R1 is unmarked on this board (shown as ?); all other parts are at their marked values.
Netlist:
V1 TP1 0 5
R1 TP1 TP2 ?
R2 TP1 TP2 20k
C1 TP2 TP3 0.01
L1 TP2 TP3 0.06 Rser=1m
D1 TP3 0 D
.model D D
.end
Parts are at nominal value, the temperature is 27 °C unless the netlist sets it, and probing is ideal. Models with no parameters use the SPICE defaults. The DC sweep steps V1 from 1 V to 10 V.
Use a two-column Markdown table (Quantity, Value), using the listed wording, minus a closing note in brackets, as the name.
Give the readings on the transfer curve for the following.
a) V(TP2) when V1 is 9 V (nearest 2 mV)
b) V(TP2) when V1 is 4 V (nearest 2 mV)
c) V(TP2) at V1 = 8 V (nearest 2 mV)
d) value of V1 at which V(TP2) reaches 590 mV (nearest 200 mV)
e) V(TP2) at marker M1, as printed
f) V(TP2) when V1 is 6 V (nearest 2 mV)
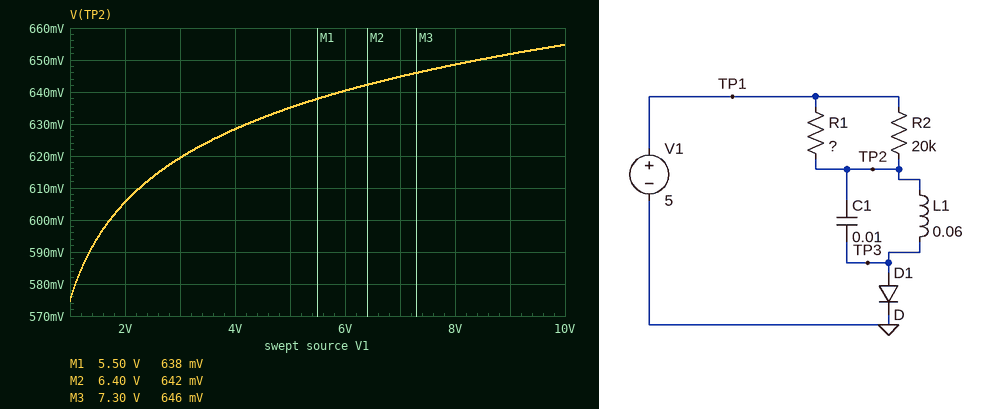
| Quantity | Value |
|---|---|
| V(TP2) when V1 is 9 V | 652 mV |
| V(TP2) when V1 is 4 V | 628 mV |
| V(TP2) at V1 = 8 V | 648 mV |
| value of V1 at which V(TP2) reaches 590 mV | 1.4 V |
| V(TP2) at marker M1, as printed | 638 mV |
| V(TP2) when V1 is 6 V | 640 mV |
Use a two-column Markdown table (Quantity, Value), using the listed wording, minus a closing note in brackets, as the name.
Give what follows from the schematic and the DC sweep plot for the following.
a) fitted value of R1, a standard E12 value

| Quantity | Value |
|---|---|
| fitted value of R1, a standard E12 value | 18 kΩ |
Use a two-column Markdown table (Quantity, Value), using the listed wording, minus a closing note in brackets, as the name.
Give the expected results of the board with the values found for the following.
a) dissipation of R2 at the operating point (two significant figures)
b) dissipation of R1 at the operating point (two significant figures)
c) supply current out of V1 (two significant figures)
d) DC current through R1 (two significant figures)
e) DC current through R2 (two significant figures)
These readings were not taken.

| Quantity | Value |
|---|---|
| dissipation of R2 at the operating point | 950 µW |
| dissipation of R1 at the operating point | 1.1 mW |
| supply current out of V1 | 460 µA |
| DC current through R1 | 240 µA |
| DC current through R2 | 220 µA |
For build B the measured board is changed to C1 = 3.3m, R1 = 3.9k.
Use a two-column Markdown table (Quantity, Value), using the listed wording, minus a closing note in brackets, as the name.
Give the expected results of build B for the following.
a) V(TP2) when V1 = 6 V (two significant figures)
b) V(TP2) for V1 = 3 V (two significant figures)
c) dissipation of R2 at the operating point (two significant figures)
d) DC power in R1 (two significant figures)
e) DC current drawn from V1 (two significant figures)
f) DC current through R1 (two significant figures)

| Quantity | Value |
|---|---|
| V(TP2) when V1 = 6 V | 670 mV |
| V(TP2) for V1 = 3 V | 650 mV |
| dissipation of R2 at the operating point | 940 µW |
| DC power in R1 | 4.8 mW |
| DC current drawn from V1 | 1.3 mA |
| DC current through R1 | 1.1 mA |
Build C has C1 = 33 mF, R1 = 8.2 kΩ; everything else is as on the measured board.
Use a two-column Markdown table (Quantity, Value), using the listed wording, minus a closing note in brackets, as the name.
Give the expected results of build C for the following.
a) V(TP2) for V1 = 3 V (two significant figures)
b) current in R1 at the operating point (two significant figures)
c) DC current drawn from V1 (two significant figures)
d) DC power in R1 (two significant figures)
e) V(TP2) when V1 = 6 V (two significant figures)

| Quantity | Value |
|---|---|
| V(TP2) for V1 = 3 V | 630 mV |
| current in R1 at the operating point | 530 µA |
| DC current drawn from V1 | 750 µA |
| DC power in R1 | 2.3 mW |
| V(TP2) when V1 = 6 V | 650 mV |
